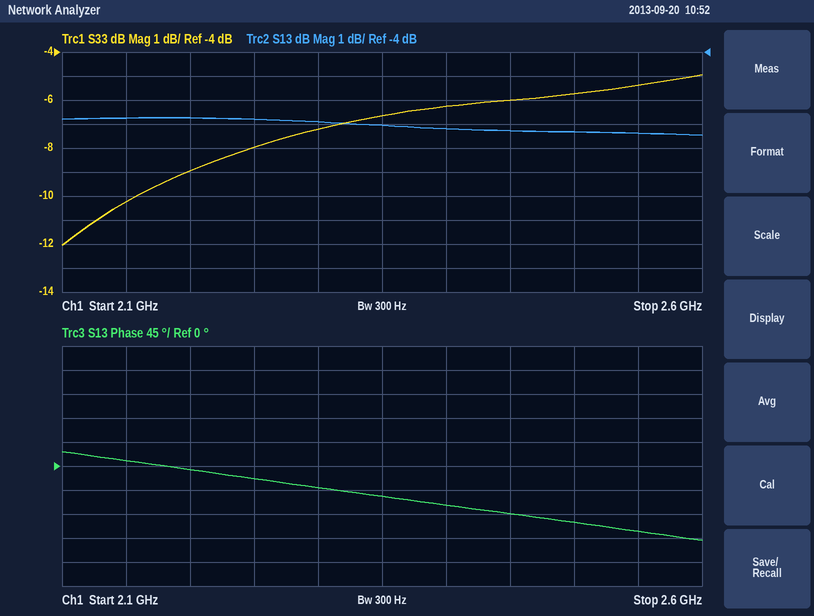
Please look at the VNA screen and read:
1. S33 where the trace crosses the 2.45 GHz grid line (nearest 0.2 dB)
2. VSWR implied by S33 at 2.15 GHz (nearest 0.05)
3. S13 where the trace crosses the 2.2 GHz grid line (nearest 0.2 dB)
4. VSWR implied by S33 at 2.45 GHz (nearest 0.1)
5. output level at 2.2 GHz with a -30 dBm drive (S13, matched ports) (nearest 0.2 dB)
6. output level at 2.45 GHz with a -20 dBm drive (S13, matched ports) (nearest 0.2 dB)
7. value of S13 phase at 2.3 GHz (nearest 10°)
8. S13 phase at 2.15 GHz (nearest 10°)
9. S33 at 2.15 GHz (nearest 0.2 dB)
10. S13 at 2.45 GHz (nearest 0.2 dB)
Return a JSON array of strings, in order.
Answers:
["-6.0 dB", "1.90", "-6.8 dB", "3.0", "-36.8 dBm", "-27.2 dBm", "-40°", "10°", "-10.2 dB", "-7.2 dB"]
